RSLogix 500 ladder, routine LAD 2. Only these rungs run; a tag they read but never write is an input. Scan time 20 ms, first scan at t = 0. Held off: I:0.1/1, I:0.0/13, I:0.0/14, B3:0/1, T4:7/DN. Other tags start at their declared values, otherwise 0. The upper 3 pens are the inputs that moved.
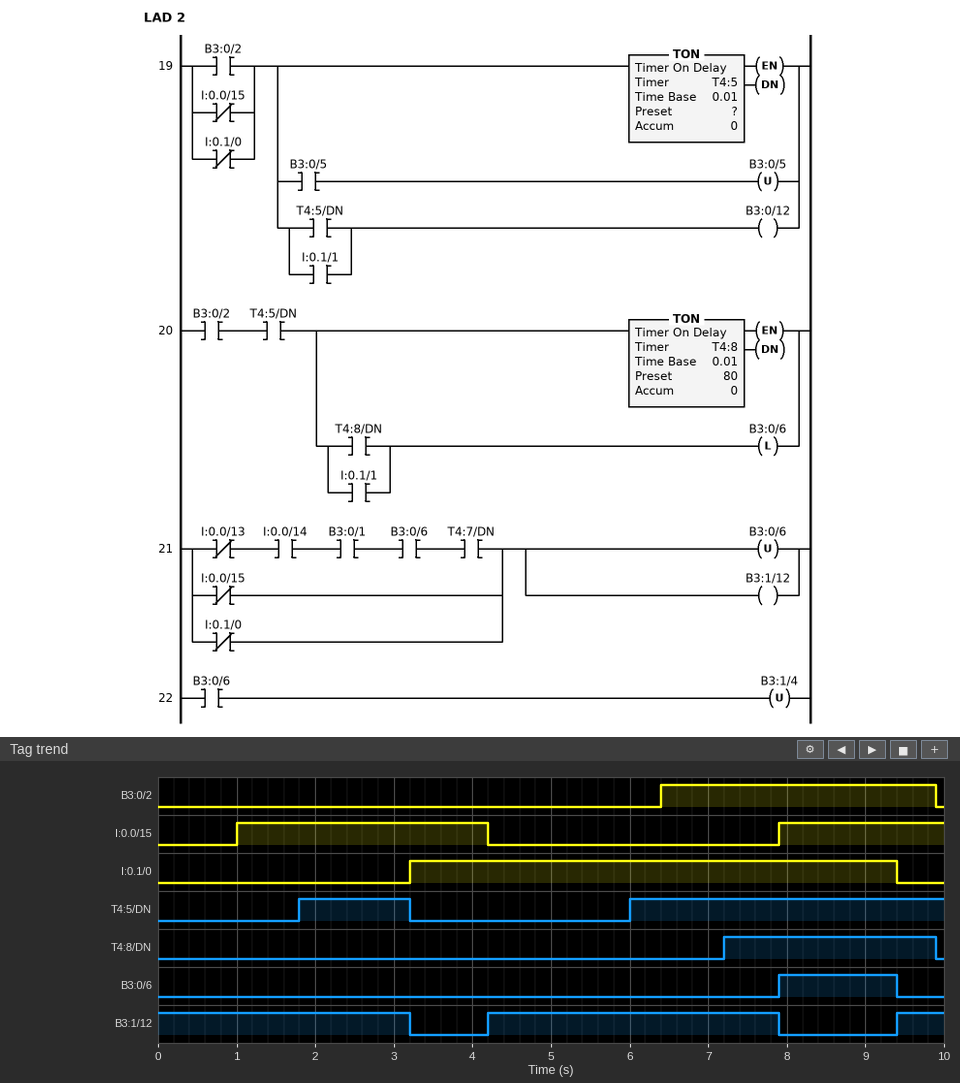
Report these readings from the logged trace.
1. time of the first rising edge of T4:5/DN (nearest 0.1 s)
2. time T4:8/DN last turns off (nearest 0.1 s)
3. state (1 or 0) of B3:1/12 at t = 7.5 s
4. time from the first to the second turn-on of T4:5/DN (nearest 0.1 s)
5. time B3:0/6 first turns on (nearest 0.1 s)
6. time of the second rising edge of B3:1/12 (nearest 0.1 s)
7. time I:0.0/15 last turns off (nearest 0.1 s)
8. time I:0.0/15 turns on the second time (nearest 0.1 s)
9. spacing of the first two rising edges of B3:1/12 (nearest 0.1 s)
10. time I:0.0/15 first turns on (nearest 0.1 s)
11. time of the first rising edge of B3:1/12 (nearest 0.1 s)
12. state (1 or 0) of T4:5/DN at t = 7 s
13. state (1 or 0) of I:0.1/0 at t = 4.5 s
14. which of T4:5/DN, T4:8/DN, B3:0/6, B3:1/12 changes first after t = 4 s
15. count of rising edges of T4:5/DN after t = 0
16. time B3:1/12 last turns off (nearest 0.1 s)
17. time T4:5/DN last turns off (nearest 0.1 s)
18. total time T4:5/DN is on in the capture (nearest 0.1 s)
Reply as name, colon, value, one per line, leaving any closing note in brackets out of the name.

time of the first rising edge of T4:5/DN: 1.8 s
time T4:8/DN last turns off: 9.9 s
state (1 or 0) of B3:1/12 at t = 7.5 s: 1
time from the first to the second turn-on of T4:5/DN: 4.2 s
time B3:0/6 first turns on: 7.9 s
time of the second rising edge of B3:1/12: 9.4 s
time I:0.0/15 last turns off: 4.2 s
time I:0.0/15 turns on the second time: 7.9 s
spacing of the first two rising edges of B3:1/12: 5.2 s
time I:0.0/15 first turns on: 1.0 s
time of the first rising edge of B3:1/12: 4.2 s
state (1 or 0) of T4:5/DN at t = 7 s: 1
state (1 or 0) of I:0.1/0 at t = 4.5 s: 1
which of T4:5/DN, T4:8/DN, B3:0/6, B3:1/12 changes first after t = 4 s: B3:1/12
count of rising edges of T4:5/DN after t = 0: 2
time B3:1/12 last turns off: 7.9 s
time T4:5/DN last turns off: 3.2 s
total time T4:5/DN is on in the capture: 5.4 s
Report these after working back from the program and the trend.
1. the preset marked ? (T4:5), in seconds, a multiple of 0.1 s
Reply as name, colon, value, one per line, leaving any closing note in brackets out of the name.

the preset marked ? (T4:5), in seconds, a multiple of 0.1 s: 1.8 s
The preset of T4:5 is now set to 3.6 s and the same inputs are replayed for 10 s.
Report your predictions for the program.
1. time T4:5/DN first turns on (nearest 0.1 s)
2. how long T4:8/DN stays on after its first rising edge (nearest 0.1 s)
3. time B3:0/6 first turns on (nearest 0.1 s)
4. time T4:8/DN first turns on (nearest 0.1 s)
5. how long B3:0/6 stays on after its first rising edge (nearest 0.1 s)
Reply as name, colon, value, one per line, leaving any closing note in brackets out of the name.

time T4:5/DN first turns on: 7.8 s
how long T4:8/DN stays on after its first rising edge: 1.3 s
time B3:0/6 first turns on: 8.6 s
time T4:8/DN first turns on: 8.6 s
how long B3:0/6 stays on after its first rising edge: 0.8 s
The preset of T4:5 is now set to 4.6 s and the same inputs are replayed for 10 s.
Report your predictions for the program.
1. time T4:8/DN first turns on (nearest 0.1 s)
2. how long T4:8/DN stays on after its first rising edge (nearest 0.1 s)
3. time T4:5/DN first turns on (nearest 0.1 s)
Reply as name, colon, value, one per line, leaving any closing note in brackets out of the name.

time T4:8/DN first turns on: 9.6 s
how long T4:8/DN stays on after its first rising edge: 0.3 s
time T4:5/DN first turns on: 8.8 s
